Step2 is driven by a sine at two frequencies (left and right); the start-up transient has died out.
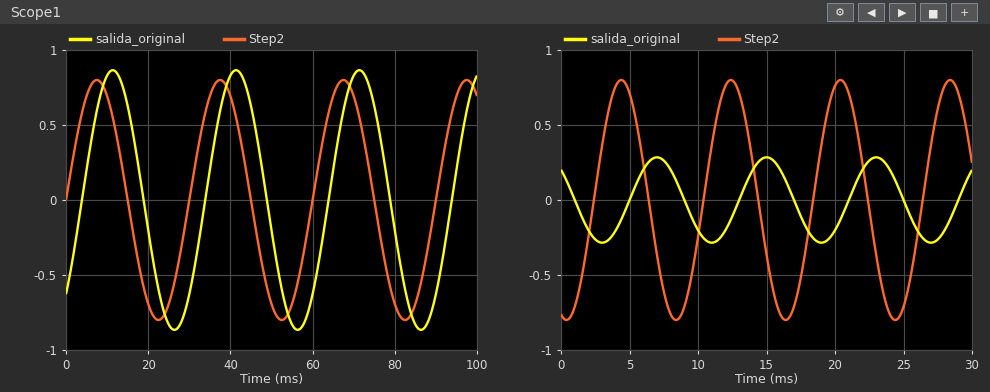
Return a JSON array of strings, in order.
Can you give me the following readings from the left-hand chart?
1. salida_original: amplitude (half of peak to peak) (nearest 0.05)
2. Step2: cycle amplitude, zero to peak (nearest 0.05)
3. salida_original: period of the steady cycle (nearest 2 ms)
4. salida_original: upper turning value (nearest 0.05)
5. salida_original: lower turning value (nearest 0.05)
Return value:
["0.85", "0.80", "30 ms", "0.85", "-0.85"]
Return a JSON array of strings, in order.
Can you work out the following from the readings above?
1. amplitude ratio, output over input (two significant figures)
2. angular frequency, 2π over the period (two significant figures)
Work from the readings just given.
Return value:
["1.1", "0.21 rad/ms"]
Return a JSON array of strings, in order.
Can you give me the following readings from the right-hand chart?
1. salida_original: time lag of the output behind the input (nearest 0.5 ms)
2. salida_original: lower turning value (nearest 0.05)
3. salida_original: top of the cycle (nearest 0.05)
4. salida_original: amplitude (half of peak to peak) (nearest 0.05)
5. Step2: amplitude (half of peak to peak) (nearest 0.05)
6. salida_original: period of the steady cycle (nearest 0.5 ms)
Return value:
["2.5 ms", "-0.30", "0.30", "0.30", "0.80", "8.0 ms"]
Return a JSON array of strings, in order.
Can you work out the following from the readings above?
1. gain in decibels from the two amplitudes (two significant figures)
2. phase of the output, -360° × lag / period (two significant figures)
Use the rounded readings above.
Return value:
["-8.5 dB", "-110°"]
